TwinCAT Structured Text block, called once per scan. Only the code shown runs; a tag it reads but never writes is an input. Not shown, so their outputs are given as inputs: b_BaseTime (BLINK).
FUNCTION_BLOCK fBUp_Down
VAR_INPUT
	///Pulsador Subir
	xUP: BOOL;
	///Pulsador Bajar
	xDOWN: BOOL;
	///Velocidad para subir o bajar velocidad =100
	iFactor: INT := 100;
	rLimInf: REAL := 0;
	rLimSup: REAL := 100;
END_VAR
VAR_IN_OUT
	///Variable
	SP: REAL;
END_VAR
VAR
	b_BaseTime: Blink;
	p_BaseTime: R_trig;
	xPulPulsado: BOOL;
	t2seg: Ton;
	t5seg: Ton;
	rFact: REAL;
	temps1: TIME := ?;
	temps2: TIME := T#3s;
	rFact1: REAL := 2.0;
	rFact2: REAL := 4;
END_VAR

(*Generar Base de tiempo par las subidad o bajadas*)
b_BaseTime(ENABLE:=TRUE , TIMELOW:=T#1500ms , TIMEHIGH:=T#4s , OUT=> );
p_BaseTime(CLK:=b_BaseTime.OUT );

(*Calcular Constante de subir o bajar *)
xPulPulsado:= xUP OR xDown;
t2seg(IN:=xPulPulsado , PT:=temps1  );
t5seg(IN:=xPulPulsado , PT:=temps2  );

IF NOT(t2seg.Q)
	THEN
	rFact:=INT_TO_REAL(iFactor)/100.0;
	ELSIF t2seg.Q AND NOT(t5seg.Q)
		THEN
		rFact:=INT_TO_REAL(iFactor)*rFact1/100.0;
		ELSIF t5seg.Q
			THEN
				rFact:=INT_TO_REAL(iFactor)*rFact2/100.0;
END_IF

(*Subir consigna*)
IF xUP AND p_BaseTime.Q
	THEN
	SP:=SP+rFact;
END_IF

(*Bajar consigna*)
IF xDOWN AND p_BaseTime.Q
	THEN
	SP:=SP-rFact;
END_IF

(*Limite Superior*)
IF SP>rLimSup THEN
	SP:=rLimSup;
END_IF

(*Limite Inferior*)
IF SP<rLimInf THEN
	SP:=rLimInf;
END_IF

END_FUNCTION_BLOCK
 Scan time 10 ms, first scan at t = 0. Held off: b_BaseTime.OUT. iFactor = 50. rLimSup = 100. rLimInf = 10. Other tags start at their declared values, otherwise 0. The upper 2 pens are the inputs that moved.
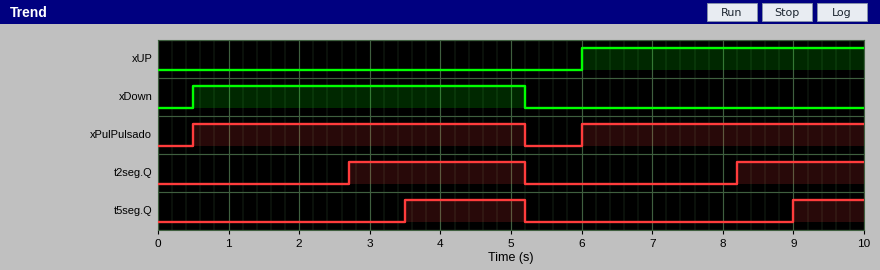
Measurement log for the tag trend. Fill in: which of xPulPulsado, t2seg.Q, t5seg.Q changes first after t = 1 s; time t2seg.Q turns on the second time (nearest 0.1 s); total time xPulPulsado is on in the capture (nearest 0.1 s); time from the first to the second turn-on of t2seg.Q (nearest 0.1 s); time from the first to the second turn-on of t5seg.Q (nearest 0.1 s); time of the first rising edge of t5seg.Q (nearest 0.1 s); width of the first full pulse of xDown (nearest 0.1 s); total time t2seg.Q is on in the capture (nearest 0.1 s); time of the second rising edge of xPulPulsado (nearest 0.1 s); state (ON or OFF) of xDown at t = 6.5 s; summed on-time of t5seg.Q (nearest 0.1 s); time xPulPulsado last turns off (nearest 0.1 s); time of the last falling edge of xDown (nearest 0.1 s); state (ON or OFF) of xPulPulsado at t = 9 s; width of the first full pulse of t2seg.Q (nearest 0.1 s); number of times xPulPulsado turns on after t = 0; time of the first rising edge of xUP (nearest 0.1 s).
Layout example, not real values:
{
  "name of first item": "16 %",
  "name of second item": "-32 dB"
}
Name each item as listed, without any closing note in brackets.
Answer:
{
  "which of xPulPulsado, t2seg.Q, t5seg.Q changes first after t = 1 s": "t2seg.Q",
  "time t2seg.Q turns on the second time": "8.2 s",
  "total time xPulPulsado is on in the capture": "8.7 s",
  "time from the first to the second turn-on of t2seg.Q": "5.5 s",
  "time from the first to the second turn-on of t5seg.Q": "5.5 s",
  "time of the first rising edge of t5seg.Q": "3.5 s",
  "width of the first full pulse of xDown": "4.7 s",
  "total time t2seg.Q is on in the capture": "4.3 s",
  "time of the second rising edge of xPulPulsado": "6.0 s",
  "state (ON or OFF) of xDown at t = 6.5 s": "OFF",
  "summed on-time of t5seg.Q": "2.7 s",
  "time xPulPulsado last turns off": "5.2 s",
  "time of the last falling edge of xDown": "5.2 s",
  "state (ON or OFF) of xPulPulsado at t = 9 s": "ON",
  "width of the first full pulse of t2seg.Q": "2.5 s",
  "number of times xPulPulsado turns on after t = 0": "2",
  "time of the first rising edge of xUP": "6.0 s"
}
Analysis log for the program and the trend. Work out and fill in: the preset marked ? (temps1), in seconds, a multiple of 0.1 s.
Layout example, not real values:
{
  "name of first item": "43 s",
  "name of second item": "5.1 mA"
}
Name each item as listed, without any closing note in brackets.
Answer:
{
  "the preset marked ? (temps1), in seconds, a multiple of 0.1 s": "2.2 s"
}
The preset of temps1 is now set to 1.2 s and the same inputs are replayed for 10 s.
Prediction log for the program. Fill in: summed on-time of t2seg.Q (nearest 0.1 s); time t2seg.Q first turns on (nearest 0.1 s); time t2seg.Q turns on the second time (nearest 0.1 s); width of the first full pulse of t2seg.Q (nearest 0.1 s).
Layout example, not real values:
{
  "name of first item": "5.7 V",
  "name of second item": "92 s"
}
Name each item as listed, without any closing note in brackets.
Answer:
{
  "summed on-time of t2seg.Q": "6.3 s",
  "time t2seg.Q first turns on": "1.7 s",
  "time t2seg.Q turns on the second time": "7.2 s",
  "width of the first full pulse of t2seg.Q": "3.5 s"
}
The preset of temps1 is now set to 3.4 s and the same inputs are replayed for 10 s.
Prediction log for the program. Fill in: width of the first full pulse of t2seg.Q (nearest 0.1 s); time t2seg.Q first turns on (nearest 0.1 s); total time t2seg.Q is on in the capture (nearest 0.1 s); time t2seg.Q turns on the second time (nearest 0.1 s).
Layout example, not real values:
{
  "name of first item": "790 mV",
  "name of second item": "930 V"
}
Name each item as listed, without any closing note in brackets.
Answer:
{
  "width of the first full pulse of t2seg.Q": "1.3 s",
  "time t2seg.Q first turns on": "3.9 s",
  "total time t2seg.Q is on in the capture": "1.9 s",
  "time t2seg.Q turns on the second time": "9.4 s"
}
